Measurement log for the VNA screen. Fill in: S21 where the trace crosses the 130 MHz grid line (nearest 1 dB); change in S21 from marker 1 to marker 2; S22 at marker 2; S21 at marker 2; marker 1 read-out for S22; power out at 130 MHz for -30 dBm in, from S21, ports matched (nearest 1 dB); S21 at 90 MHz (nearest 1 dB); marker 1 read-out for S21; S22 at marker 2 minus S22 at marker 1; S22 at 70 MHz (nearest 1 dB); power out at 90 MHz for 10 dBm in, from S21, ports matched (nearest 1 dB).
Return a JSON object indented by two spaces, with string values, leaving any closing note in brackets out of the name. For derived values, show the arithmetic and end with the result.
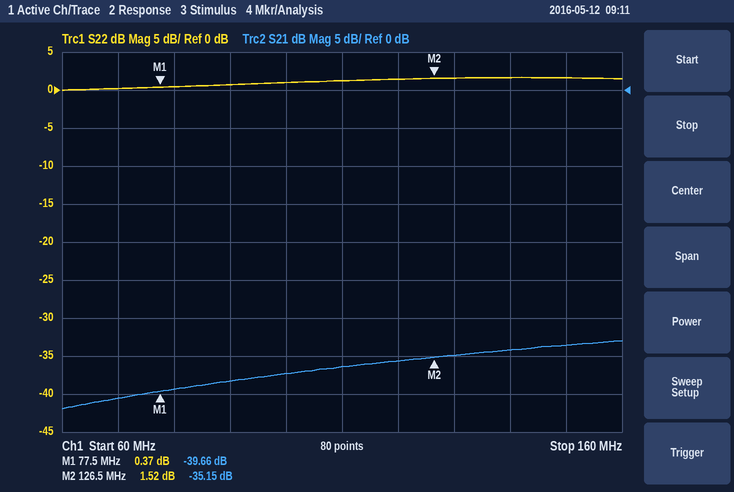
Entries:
{
  "S21 where the trace crosses the 130 MHz grid line": "-35 dB",
  "change in S21 from marker 1 to marker 2": "-35.15 − (-39.66) = 4.51 dB",
  "S22 at marker 2": "1.52 dB",
  "S21 at marker 2": "-35.15 dB",
  "marker 1 read-out for S22": "0.37 dB",
  "power out at 130 MHz for -30 dBm in, from S21, ports matched": "-30 dBm + (-35 dB) = -65 dBm",
  "S21 at 90 MHz": "-38 dB",
  "marker 1 read-out for S21": "-39.66 dB",
  "S22 at marker 2 minus S22 at marker 1": "1.52 − (0.37) = 1.15 dB",
  "S22 at 70 MHz": "0 dB",
  "power out at 90 MHz for 10 dBm in, from S21, ports matched": "10 dBm + (-38 dB) = -28 dBm"
}
